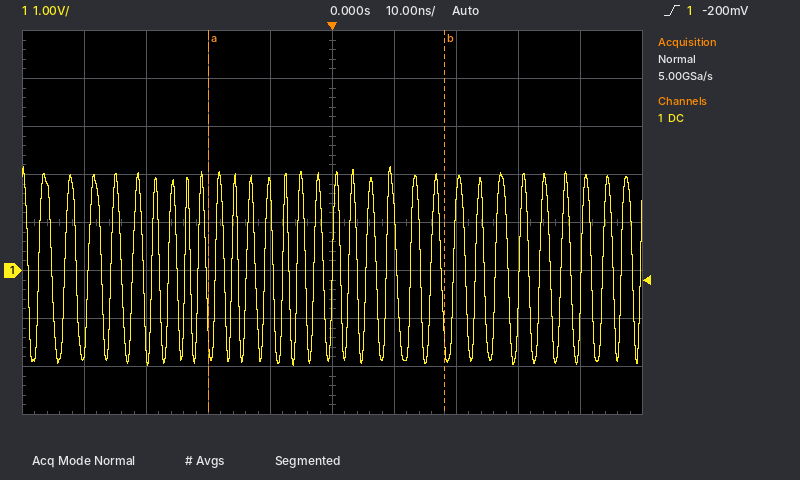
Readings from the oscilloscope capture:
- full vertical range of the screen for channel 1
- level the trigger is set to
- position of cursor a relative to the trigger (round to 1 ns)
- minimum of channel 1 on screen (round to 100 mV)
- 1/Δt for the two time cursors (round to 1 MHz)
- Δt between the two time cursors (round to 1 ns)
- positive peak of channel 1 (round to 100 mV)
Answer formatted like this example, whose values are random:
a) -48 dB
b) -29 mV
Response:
a) 8 V
b) -200 mV
c) -20 ns
d) -2.0 V
e) 26 MHz
f) 38 ns
g) 2.2 V
